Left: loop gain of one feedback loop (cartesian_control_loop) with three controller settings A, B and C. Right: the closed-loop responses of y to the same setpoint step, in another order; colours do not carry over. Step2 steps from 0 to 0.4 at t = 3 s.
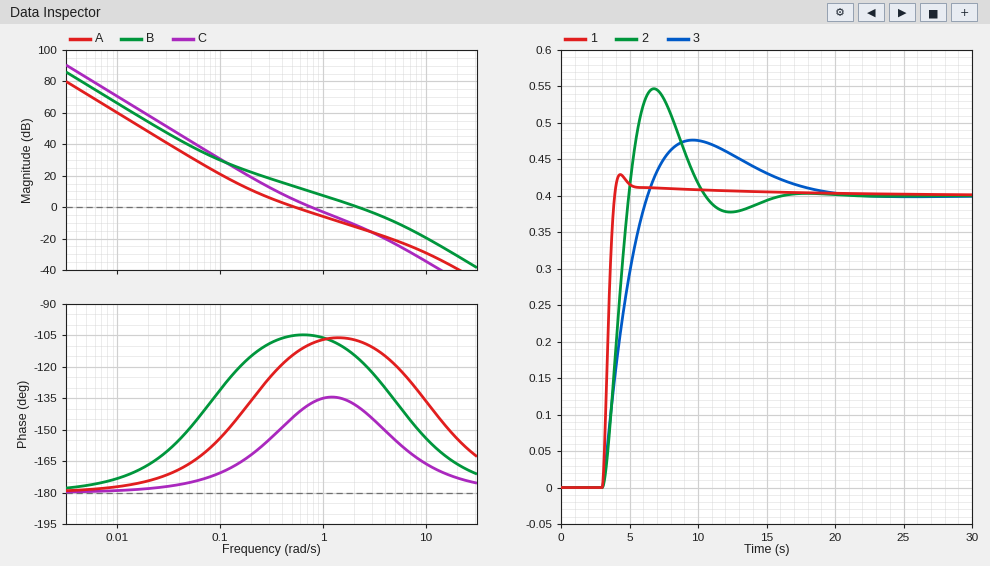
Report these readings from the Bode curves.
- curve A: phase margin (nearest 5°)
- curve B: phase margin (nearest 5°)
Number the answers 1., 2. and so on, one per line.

1. 65°
2. 65°
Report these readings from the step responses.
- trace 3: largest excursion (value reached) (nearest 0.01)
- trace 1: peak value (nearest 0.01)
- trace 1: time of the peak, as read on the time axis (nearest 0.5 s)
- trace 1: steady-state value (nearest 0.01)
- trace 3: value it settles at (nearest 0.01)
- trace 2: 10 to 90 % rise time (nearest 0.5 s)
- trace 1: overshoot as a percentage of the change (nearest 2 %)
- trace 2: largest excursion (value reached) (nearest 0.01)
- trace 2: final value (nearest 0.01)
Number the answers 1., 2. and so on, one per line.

1. 0.48
2. 0.43
3. 4.5 s
4. 0.40
5. 0.40
6. 1.5 s
7. 8 %
8. 0.55
9. 0.40
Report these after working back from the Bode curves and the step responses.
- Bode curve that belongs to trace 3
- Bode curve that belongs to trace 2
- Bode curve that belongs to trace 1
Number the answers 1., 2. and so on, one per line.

1. A
2. C
3. B
